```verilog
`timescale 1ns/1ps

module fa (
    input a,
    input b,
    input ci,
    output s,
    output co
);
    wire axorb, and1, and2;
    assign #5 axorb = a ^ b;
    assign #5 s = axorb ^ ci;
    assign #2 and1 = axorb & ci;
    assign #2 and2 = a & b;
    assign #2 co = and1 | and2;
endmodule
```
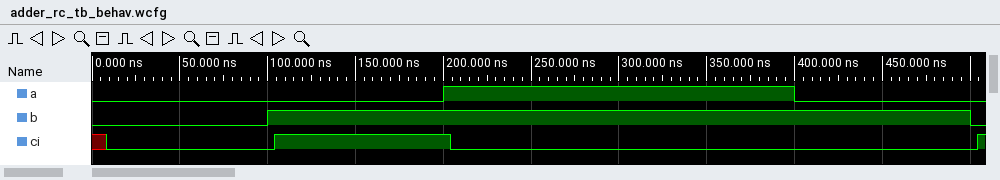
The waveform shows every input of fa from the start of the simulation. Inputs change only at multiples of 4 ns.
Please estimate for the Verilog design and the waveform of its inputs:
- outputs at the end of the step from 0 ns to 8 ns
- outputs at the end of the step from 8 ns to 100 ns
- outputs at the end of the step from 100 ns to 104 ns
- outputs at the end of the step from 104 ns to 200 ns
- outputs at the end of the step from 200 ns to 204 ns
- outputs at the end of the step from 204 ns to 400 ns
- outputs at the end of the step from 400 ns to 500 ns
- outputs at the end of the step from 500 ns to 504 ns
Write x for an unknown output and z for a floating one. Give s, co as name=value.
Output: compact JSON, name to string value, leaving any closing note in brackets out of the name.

{"outputs at the end of the step from 0 ns to 8 ns": "s=x, co=x", "outputs at the end of the step from 8 ns to 100 ns": "s=0, co=0", "outputs at the end of the step from 100 ns to 104 ns": "s=0, co=0", "outputs at the end of the step from 104 ns to 200 ns": "s=0, co=1", "outputs at the end of the step from 200 ns to 204 ns": "s=0, co=1", "outputs at the end of the step from 204 ns to 400 ns": "s=0, co=1", "outputs at the end of the step from 400 ns to 500 ns": "s=1, co=0", "outputs at the end of the step from 500 ns to 504 ns": "s=1, co=0"}
